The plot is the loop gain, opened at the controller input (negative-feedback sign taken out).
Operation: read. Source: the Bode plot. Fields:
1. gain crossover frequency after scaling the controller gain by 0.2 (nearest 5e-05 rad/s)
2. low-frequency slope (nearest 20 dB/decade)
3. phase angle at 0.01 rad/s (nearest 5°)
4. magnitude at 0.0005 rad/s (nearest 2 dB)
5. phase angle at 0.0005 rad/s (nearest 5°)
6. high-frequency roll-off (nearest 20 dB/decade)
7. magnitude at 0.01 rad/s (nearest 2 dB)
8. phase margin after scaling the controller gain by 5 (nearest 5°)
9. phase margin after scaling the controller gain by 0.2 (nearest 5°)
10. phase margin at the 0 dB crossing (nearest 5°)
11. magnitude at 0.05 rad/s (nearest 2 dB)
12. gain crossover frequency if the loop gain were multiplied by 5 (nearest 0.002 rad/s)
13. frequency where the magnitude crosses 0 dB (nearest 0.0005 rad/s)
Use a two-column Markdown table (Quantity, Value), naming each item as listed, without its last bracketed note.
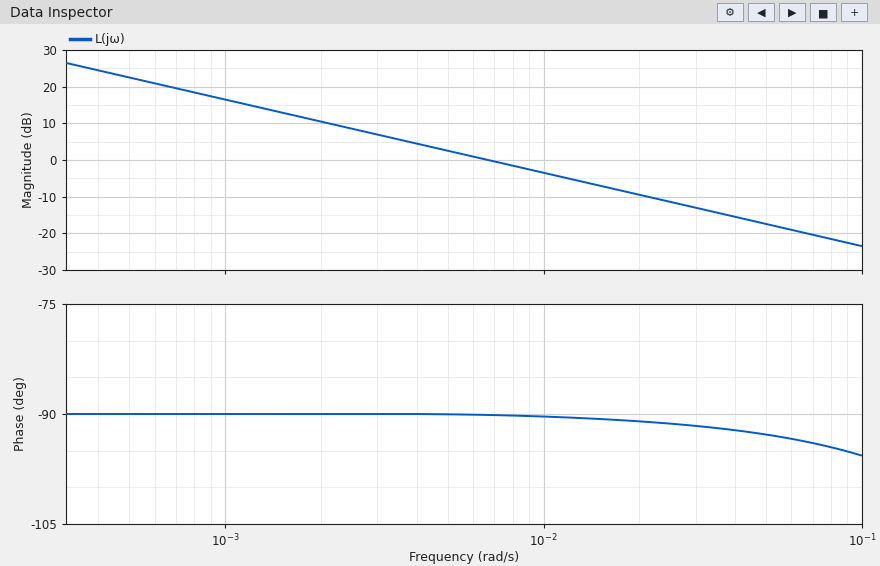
| Quantity | Value |
|---|---|
| gain crossover frequency after scaling the controller gain by 0.2 | 0.00135 rad/s |
| low-frequency slope | -20 dB/decade |
| phase angle at 0.01 rad/s | -90° |
| magnitude at 0.0005 rad/s | 22 dB |
| phase angle at 0.0005 rad/s | -90° |
| high-frequency roll-off | -20 dB/decade |
| magnitude at 0.01 rad/s | -4 dB |
| phase margin after scaling the controller gain by 5 | 90° |
| phase margin after scaling the controller gain by 0.2 | 90° |
| phase margin at the 0 dB crossing | 90° |
| magnitude at 0.05 rad/s | -18 dB |
| gain crossover frequency if the loop gain were multiplied by 5 | 0.034 rad/s |
| frequency where the magnitude crosses 0 dB | 0.0065 rad/s |
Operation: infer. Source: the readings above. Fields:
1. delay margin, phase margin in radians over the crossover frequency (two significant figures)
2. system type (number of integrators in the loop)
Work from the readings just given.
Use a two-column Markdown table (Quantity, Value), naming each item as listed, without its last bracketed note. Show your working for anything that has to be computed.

| Quantity | Value |
|---|---|
| delay margin, phase margin in radians over the crossover frequency | 90 × π / 180 / 0.0065 = 240 s |
| system type | 1 |
